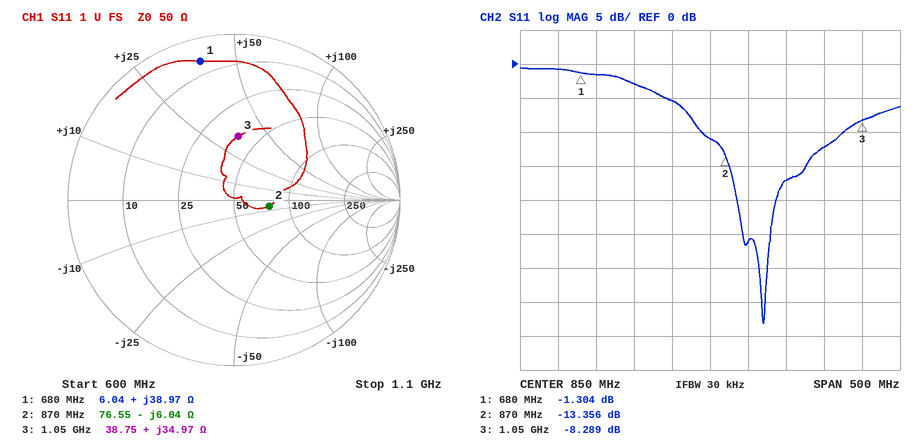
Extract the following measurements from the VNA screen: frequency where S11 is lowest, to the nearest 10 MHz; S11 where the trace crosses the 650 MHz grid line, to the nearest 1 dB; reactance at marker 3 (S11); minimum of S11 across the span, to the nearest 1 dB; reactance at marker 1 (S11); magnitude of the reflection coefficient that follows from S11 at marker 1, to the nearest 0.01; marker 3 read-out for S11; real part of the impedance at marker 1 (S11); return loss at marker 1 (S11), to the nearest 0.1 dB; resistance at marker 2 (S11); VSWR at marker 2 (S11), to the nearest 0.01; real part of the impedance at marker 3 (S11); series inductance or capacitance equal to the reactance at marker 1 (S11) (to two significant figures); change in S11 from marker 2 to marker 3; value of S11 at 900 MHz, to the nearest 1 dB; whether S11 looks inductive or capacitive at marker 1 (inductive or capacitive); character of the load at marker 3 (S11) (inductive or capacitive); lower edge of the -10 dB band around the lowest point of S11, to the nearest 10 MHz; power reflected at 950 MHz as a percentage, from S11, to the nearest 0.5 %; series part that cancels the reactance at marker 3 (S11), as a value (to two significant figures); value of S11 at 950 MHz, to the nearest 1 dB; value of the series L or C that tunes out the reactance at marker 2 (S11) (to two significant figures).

920 MHz
-1 dB
+34.97 Ω
-38 dB
+38.97 Ω
0.86
-8.289 dB
6.04 Ω
1.3 dB
76.55 Ω
1.55
38.75 Ω
9.1 nH
5.067 dB
-26 dB
inductive
inductive
840 MHz
2.0 %
4.3 pF
-17 dB
1.1 nH
